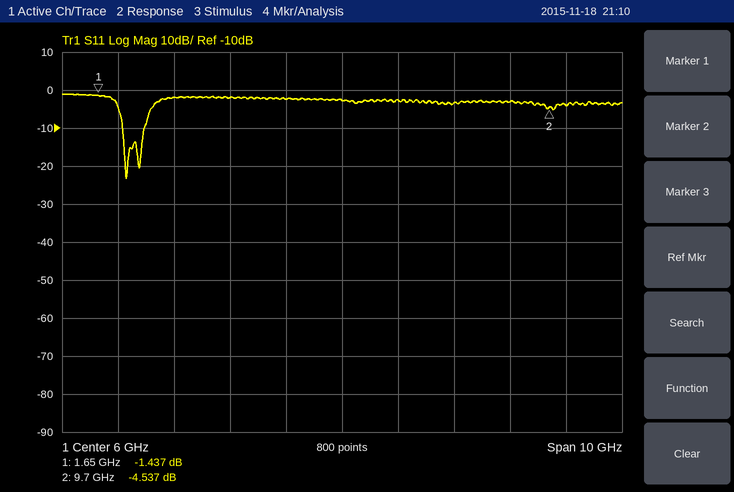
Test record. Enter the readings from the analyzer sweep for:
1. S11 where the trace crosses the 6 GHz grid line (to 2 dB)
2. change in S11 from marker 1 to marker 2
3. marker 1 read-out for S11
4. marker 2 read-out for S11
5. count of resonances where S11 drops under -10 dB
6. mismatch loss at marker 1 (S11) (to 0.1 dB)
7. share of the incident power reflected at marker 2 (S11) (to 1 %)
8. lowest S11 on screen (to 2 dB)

-2 dB
-3.100 dB
-1.437 dB
-4.537 dB
2
5.5 dB
35 %
-24 dB
